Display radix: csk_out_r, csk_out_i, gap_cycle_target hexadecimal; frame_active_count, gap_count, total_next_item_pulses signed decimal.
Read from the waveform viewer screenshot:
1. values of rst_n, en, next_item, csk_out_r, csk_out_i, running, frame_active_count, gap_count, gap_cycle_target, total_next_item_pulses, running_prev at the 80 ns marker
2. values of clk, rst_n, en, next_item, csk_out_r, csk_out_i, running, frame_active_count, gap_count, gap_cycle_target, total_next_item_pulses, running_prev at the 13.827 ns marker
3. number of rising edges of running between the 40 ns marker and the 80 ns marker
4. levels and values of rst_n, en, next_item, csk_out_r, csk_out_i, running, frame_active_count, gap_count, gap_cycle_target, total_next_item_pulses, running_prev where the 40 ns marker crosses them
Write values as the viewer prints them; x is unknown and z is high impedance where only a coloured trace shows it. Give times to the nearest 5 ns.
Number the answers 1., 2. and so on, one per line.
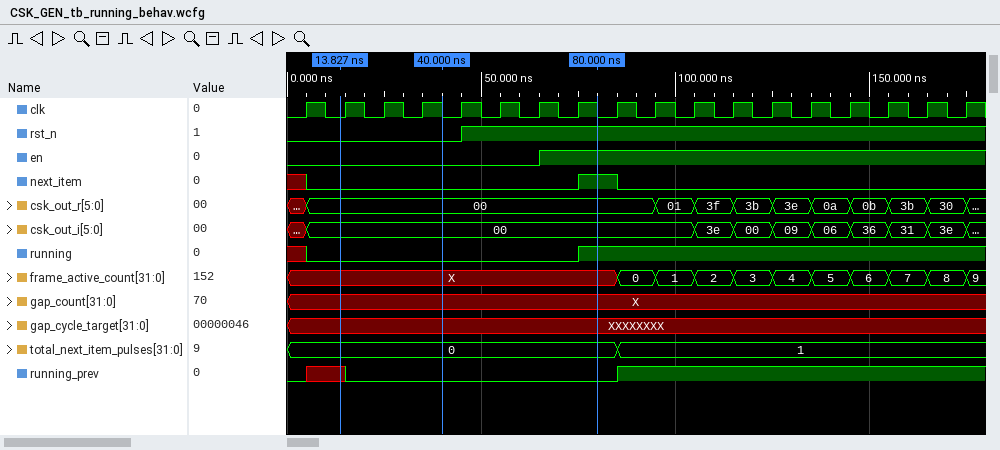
1. rst_n=1, en=1, next_item=1, csk_out_r=00, csk_out_i=00, running=1, frame_active_count=X, gap_count=X, gap_cycle_target=XXXXXXXX, total_next_item_pulses=0, running_prev=0
2. clk=0, rst_n=0, en=0, next_item=0, csk_out_r=00, csk_out_i=00, running=0, frame_active_count=X, gap_count=X, gap_cycle_target=XXXXXXXX, total_next_item_pulses=0, running_prev=x
3. 1
4. rst_n=0, en=0, next_item=0, csk_out_r=00, csk_out_i=00, running=0, frame_active_count=X, gap_count=X, gap_cycle_target=XXXXXXXX, total_next_item_pulses=0, running_prev=0
